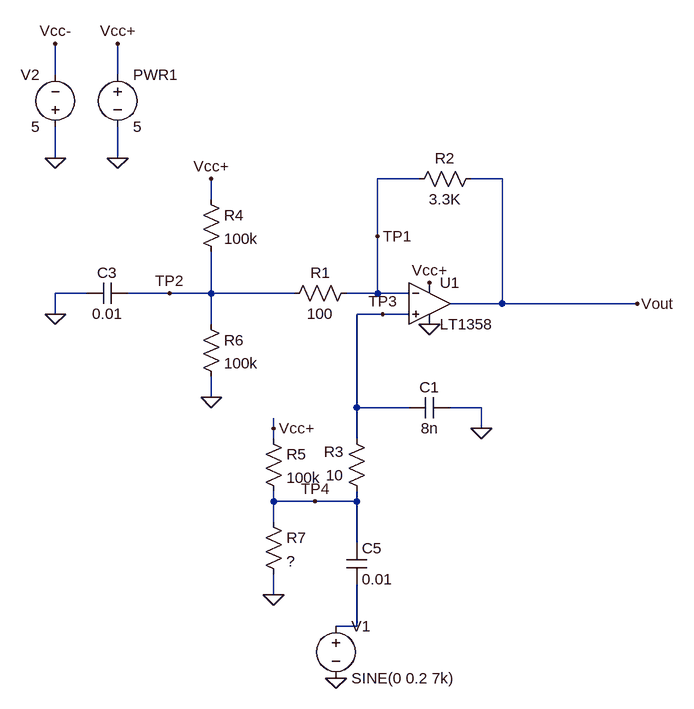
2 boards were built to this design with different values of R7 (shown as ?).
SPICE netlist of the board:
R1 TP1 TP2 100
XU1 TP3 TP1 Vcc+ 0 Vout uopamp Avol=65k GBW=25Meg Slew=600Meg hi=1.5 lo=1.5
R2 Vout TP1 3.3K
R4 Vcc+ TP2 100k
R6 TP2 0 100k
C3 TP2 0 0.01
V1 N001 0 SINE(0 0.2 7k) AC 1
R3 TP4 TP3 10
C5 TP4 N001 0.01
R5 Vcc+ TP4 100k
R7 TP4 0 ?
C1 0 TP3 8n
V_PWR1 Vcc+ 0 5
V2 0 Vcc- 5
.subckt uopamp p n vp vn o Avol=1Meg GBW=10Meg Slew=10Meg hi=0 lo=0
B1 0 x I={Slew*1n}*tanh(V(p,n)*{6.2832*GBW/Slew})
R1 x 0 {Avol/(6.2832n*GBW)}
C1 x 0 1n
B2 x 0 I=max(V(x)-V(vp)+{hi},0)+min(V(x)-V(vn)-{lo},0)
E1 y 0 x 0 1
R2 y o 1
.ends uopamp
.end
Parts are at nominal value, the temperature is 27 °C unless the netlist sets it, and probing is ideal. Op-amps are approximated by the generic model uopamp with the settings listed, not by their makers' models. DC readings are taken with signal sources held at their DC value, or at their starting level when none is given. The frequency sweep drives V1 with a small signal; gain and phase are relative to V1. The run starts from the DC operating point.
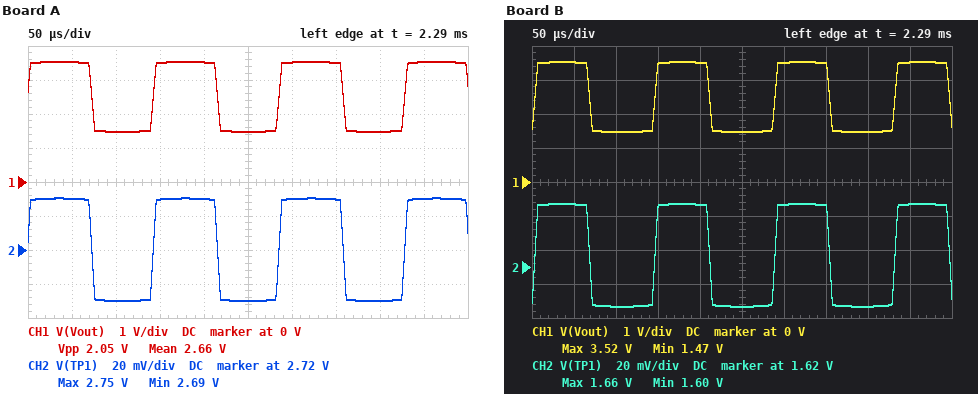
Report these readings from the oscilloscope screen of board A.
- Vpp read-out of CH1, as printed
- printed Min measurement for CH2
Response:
2.05 V
2.69 V
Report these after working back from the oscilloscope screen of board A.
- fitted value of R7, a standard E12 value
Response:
120 kΩ
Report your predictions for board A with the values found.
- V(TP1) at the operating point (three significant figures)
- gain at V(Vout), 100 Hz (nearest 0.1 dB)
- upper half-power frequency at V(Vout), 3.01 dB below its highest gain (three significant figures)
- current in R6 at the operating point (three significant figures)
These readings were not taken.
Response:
2.73 V
30.6 dB
659 kHz
27.3 µA
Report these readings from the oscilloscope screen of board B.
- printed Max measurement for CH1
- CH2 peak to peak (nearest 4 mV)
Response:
3.52 V
60 mV
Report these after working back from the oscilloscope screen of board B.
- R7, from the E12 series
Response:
47 kΩ
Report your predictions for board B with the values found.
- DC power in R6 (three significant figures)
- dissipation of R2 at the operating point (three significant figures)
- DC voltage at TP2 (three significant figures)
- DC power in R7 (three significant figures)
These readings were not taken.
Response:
25.6 µW
1.07 µW
1.60 V
54.4 µW
